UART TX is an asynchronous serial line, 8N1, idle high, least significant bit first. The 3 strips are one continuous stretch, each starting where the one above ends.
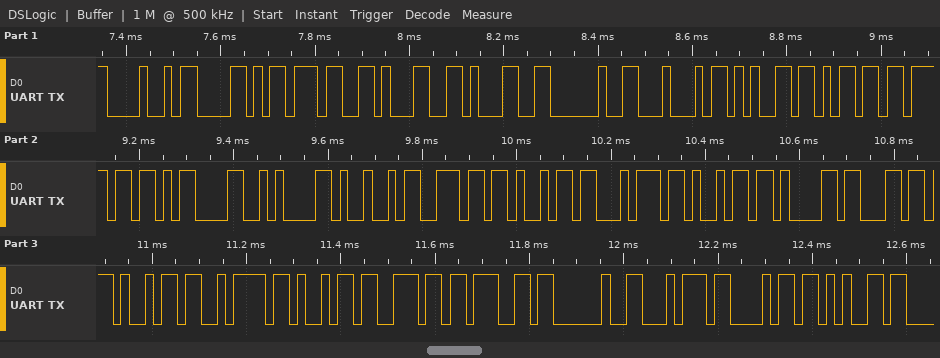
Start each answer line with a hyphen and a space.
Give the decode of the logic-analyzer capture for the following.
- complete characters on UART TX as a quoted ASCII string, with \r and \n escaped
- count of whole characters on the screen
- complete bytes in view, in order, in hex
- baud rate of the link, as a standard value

- "HX711 Demo\r\nInitializing the"
- 28
- 48 58 37 31 31 20 44 65 6D 6F 0D 0A 49 6E 69 74 69 61 6C 69 7A 69 6E 67 20 74 68 65
- 57600 baud
